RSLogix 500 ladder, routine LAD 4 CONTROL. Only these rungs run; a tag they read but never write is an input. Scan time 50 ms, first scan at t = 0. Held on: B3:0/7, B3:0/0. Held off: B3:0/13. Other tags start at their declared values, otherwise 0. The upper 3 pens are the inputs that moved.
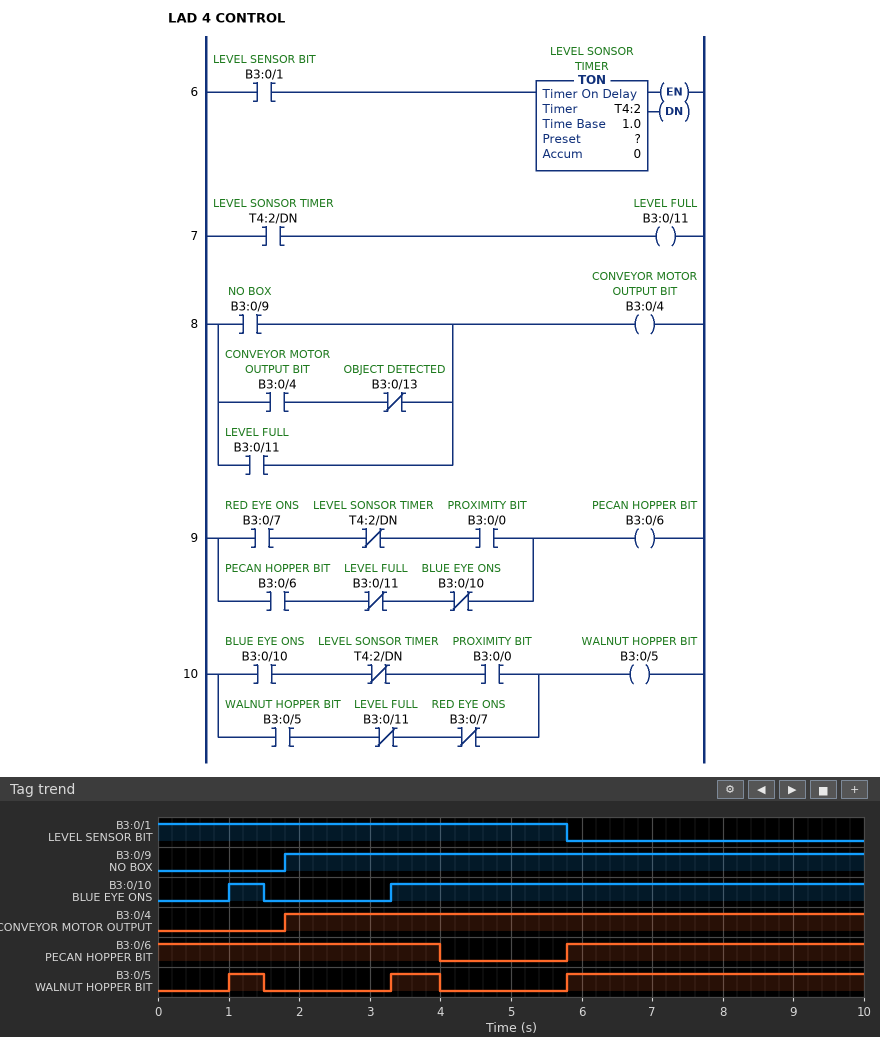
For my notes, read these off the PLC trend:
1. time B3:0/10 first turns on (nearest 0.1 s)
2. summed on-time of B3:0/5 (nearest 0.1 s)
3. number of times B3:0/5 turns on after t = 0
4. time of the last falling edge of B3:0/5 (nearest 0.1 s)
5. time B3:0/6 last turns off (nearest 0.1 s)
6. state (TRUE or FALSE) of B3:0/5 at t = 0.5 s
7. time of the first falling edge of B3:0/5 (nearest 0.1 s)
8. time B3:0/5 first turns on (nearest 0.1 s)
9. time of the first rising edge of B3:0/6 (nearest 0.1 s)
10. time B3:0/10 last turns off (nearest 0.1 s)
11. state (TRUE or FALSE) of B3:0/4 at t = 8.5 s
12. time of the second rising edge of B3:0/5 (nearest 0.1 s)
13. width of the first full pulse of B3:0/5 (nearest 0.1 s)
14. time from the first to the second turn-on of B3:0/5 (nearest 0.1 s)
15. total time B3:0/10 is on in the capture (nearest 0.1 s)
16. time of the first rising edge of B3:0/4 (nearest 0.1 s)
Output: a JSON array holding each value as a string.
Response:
["1.0 s", "5.4 s", "3", "4.0 s", "4.0 s", "FALSE", "1.5 s", "1.0 s", "5.8 s", "1.5 s", "TRUE", "3.3 s", "0.5 s", "2.3 s", "7.2 s", "1.8 s"]
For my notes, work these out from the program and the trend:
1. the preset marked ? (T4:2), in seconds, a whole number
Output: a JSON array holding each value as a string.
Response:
["4 s"]
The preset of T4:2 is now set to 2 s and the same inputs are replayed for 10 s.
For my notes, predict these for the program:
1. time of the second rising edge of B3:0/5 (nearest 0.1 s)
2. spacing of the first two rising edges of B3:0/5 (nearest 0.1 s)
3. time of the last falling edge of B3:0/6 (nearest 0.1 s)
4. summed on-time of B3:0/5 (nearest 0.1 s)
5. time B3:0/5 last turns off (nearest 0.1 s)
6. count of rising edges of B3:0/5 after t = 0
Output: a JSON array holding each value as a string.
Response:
["5.8 s", "4.8 s", "2.0 s", "4.7 s", "1.5 s", "2"]
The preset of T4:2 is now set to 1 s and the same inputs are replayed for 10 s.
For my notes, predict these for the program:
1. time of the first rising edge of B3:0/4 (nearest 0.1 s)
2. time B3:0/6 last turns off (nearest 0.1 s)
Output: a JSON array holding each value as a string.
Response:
["1.0 s", "1.0 s"]
